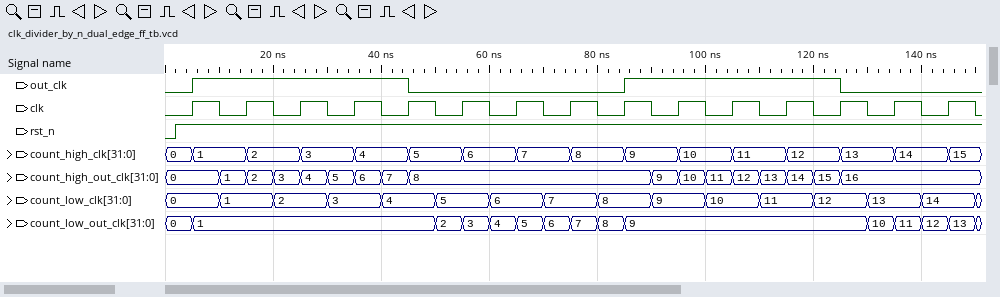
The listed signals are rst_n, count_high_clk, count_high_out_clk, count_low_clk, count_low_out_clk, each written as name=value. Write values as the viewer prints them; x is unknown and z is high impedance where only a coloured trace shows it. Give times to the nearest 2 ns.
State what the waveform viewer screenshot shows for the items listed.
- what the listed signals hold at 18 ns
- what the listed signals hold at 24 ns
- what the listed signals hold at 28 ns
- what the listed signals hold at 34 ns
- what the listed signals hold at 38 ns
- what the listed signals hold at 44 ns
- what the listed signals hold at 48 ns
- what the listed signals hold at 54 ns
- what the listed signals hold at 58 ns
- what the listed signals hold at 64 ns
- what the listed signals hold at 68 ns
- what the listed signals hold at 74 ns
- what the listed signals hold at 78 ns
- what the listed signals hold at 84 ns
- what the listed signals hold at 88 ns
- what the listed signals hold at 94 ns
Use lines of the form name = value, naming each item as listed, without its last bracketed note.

what the listed signals hold at 18 ns = rst_n=1, count_high_clk=2, count_high_out_clk=2, count_low_clk=1, count_low_out_clk=1
what the listed signals hold at 24 ns = rst_n=1, count_high_clk=2, count_high_out_clk=3, count_low_clk=2, count_low_out_clk=1
what the listed signals hold at 28 ns = rst_n=1, count_high_clk=3, count_high_out_clk=4, count_low_clk=2, count_low_out_clk=1
what the listed signals hold at 34 ns = rst_n=1, count_high_clk=3, count_high_out_clk=5, count_low_clk=3, count_low_out_clk=1
what the listed signals hold at 38 ns = rst_n=1, count_high_clk=4, count_high_out_clk=6, count_low_clk=3, count_low_out_clk=1
what the listed signals hold at 44 ns = rst_n=1, count_high_clk=4, count_high_out_clk=7, count_low_clk=4, count_low_out_clk=1
what the listed signals hold at 48 ns = rst_n=1, count_high_clk=5, count_high_out_clk=8, count_low_clk=4, count_low_out_clk=1
what the listed signals hold at 54 ns = rst_n=1, count_high_clk=5, count_high_out_clk=8, count_low_clk=5, count_low_out_clk=2
what the listed signals hold at 58 ns = rst_n=1, count_high_clk=6, count_high_out_clk=8, count_low_clk=5, count_low_out_clk=3
what the listed signals hold at 64 ns = rst_n=1, count_high_clk=6, count_high_out_clk=8, count_low_clk=6, count_low_out_clk=4
what the listed signals hold at 68 ns = rst_n=1, count_high_clk=7, count_high_out_clk=8, count_low_clk=6, count_low_out_clk=5
what the listed signals hold at 74 ns = rst_n=1, count_high_clk=7, count_high_out_clk=8, count_low_clk=7, count_low_out_clk=6
what the listed signals hold at 78 ns = rst_n=1, count_high_clk=8, count_high_out_clk=8, count_low_clk=7, count_low_out_clk=7
what the listed signals hold at 84 ns = rst_n=1, count_high_clk=8, count_high_out_clk=8, count_low_clk=8, count_low_out_clk=8
what the listed signals hold at 88 ns = rst_n=1, count_high_clk=9, count_high_out_clk=8, count_low_clk=8, count_low_out_clk=9
what the listed signals hold at 94 ns = rst_n=1, count_high_clk=9, count_high_out_clk=9, count_low_clk=9, count_low_out_clk=9
